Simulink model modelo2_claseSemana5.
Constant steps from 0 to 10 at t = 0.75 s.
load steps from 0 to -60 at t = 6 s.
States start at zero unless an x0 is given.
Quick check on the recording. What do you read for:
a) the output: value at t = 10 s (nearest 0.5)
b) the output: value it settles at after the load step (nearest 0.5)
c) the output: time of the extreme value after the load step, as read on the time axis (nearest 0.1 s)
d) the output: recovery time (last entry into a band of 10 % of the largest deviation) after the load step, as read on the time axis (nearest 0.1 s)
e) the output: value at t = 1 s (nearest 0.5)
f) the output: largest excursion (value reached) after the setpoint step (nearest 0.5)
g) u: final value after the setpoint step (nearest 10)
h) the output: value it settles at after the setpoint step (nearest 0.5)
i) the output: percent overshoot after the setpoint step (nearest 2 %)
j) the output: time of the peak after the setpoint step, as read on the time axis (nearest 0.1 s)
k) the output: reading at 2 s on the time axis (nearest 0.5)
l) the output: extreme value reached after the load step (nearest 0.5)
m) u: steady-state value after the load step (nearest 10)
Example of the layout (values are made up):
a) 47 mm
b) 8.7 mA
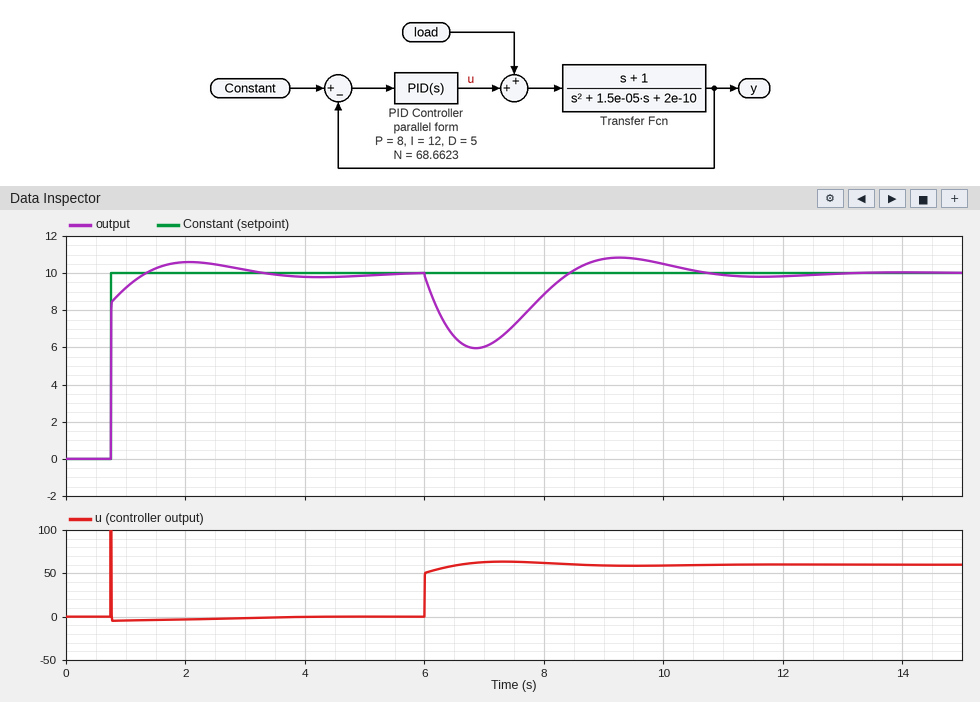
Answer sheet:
a) 10.5
b) 10.0
c) 6.9 s
d) 10.1 s
e) 9.0
f) 10.5
g) 0
h) 10.0
i) 6 %
j) 2.1 s
k) 10.5
l) 6.0
m) 60
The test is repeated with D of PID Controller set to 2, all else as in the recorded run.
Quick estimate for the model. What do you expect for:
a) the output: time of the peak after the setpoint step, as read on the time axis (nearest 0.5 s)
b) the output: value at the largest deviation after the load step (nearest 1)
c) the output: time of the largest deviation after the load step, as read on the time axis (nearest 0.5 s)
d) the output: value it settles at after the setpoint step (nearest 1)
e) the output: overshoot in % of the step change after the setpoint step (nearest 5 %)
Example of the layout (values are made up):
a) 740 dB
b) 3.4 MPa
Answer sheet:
a) 1.5 s
b) 5
c) 6.5 s
d) 10
e) 10 %
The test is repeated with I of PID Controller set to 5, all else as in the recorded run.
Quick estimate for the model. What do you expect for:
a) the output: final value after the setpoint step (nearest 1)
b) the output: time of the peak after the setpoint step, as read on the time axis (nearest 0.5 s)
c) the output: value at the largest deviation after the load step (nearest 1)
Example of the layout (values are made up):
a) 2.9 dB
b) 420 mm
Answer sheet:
a) 10
b) 2.5 s
c) 5
